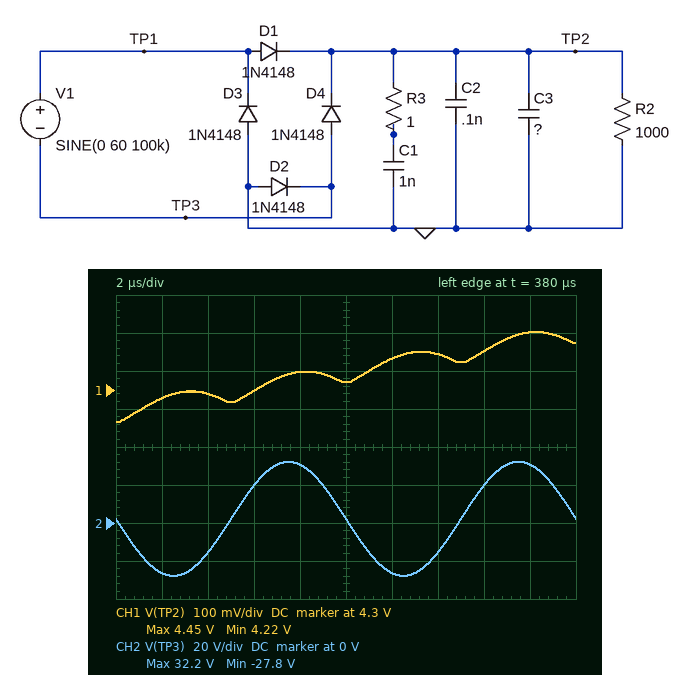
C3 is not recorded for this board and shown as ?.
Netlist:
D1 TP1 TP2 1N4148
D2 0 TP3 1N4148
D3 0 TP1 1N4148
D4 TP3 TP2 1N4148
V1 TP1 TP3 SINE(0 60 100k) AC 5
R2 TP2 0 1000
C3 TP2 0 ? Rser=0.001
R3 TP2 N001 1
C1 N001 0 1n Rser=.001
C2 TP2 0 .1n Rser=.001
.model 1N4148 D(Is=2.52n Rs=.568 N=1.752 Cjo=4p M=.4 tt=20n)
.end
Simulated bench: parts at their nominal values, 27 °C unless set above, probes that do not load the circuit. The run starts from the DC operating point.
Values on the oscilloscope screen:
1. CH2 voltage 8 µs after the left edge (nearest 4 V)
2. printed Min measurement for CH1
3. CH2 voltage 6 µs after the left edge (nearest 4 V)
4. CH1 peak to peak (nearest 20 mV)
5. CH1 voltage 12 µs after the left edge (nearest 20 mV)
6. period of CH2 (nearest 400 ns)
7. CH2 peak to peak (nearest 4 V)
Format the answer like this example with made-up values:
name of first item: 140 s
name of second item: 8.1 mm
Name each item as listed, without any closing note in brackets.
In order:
CH2 voltage 8 µs after the left edge: 32 V
printed Min measurement for CH1: 4.22 V
CH2 voltage 6 µs after the left edge: 20 V
CH1 peak to peak: 240 mV
CH1 voltage 12 µs after the left edge: 4.38 V
period of CH2: 10.0 µs
CH2 peak to peak: 60 V
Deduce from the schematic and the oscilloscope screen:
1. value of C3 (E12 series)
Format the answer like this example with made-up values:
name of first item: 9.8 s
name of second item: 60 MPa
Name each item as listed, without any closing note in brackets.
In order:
value of C3: 2.7 mF
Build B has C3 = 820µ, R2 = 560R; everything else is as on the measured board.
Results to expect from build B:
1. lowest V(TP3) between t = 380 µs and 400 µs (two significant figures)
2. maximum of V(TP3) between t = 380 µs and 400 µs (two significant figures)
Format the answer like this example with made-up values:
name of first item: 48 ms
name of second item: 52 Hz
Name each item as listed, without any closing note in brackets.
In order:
lowest V(TP3) between t = 380 µs and 400 µs: -24 V
maximum of V(TP3) between t = 380 µs and 400 µs: 36 V
